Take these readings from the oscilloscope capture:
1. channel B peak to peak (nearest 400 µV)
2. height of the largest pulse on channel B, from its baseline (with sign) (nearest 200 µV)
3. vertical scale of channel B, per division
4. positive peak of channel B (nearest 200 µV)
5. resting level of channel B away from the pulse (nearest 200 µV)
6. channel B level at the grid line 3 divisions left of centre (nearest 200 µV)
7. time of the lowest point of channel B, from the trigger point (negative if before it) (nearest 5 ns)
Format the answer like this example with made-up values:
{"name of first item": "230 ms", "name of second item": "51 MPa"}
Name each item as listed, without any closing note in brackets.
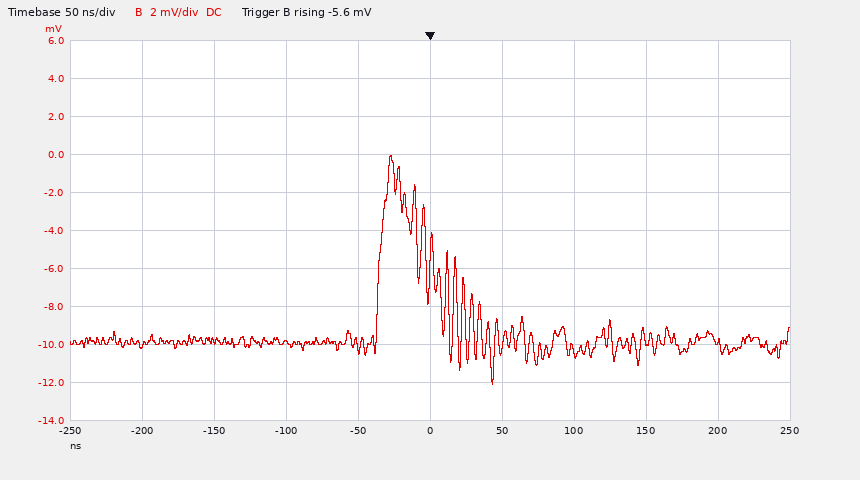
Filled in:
{"channel B peak to peak": "12.0 mV", "height of the largest pulse on channel B, from its baseline (with sign)": "+9.8 mV", "vertical scale of channel B, per division": "2 mV", "positive peak of channel B": "0.0 mV", "resting level of channel B away from the pulse": "-9.8 mV", "channel B level at the grid line 3 divisions left of centre": "-9.8 mV", "time of the lowest point of channel B, from the trigger point (negative if before it)": "+45 ns"}
